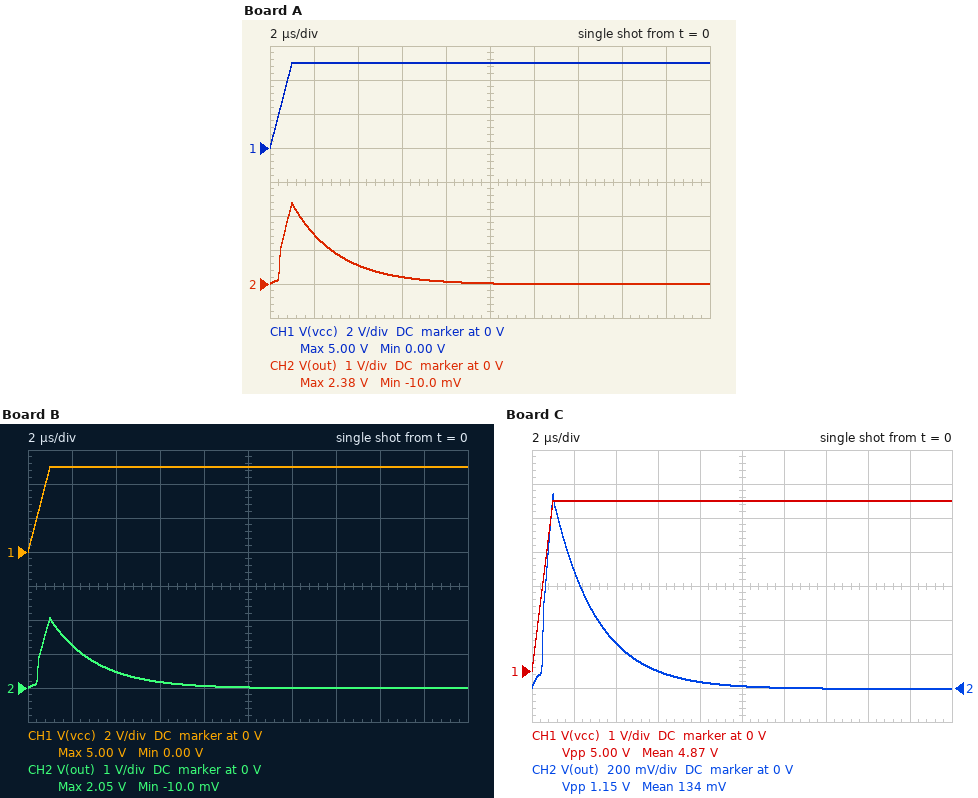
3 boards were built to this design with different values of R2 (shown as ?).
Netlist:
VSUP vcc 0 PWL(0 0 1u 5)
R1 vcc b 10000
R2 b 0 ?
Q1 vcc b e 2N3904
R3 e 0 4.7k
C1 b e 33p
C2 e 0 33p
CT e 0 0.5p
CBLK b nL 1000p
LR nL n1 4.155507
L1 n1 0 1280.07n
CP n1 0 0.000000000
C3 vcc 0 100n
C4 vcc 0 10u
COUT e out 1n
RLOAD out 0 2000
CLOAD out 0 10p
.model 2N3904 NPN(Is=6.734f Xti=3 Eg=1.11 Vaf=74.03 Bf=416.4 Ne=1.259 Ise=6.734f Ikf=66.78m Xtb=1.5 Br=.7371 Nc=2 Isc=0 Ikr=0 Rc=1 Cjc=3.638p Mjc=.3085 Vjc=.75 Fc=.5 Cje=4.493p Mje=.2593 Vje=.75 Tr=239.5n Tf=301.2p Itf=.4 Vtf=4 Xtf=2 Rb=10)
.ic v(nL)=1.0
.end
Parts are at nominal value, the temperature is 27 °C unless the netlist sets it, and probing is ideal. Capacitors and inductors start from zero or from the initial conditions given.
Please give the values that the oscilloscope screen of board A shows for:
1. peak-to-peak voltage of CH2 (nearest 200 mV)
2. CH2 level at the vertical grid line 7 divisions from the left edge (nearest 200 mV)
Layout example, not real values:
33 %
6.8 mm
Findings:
2.4 V
0 V
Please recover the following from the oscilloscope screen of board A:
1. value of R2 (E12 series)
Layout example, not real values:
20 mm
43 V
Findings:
27 kΩ
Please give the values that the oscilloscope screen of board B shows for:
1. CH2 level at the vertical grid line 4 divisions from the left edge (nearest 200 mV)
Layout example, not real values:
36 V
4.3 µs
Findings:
0 V
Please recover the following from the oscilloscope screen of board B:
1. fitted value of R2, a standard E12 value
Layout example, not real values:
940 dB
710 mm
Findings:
18 kΩ
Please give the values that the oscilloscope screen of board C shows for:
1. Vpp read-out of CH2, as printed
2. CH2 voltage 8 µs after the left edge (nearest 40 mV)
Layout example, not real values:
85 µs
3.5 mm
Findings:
1.15 V
40 mV
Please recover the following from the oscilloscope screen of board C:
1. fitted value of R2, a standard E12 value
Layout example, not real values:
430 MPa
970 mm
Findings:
6.8 kΩ
